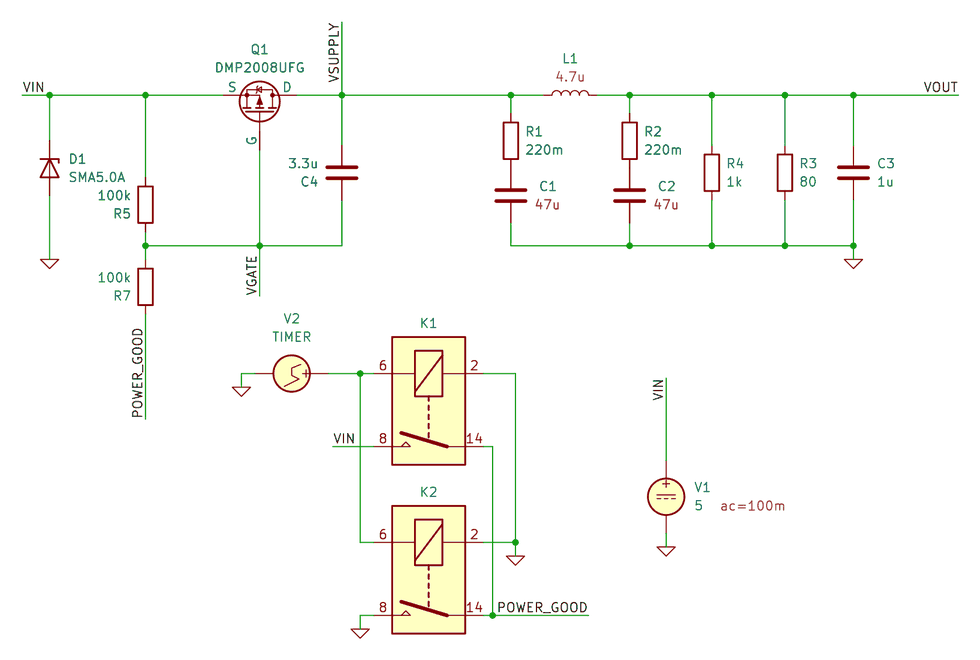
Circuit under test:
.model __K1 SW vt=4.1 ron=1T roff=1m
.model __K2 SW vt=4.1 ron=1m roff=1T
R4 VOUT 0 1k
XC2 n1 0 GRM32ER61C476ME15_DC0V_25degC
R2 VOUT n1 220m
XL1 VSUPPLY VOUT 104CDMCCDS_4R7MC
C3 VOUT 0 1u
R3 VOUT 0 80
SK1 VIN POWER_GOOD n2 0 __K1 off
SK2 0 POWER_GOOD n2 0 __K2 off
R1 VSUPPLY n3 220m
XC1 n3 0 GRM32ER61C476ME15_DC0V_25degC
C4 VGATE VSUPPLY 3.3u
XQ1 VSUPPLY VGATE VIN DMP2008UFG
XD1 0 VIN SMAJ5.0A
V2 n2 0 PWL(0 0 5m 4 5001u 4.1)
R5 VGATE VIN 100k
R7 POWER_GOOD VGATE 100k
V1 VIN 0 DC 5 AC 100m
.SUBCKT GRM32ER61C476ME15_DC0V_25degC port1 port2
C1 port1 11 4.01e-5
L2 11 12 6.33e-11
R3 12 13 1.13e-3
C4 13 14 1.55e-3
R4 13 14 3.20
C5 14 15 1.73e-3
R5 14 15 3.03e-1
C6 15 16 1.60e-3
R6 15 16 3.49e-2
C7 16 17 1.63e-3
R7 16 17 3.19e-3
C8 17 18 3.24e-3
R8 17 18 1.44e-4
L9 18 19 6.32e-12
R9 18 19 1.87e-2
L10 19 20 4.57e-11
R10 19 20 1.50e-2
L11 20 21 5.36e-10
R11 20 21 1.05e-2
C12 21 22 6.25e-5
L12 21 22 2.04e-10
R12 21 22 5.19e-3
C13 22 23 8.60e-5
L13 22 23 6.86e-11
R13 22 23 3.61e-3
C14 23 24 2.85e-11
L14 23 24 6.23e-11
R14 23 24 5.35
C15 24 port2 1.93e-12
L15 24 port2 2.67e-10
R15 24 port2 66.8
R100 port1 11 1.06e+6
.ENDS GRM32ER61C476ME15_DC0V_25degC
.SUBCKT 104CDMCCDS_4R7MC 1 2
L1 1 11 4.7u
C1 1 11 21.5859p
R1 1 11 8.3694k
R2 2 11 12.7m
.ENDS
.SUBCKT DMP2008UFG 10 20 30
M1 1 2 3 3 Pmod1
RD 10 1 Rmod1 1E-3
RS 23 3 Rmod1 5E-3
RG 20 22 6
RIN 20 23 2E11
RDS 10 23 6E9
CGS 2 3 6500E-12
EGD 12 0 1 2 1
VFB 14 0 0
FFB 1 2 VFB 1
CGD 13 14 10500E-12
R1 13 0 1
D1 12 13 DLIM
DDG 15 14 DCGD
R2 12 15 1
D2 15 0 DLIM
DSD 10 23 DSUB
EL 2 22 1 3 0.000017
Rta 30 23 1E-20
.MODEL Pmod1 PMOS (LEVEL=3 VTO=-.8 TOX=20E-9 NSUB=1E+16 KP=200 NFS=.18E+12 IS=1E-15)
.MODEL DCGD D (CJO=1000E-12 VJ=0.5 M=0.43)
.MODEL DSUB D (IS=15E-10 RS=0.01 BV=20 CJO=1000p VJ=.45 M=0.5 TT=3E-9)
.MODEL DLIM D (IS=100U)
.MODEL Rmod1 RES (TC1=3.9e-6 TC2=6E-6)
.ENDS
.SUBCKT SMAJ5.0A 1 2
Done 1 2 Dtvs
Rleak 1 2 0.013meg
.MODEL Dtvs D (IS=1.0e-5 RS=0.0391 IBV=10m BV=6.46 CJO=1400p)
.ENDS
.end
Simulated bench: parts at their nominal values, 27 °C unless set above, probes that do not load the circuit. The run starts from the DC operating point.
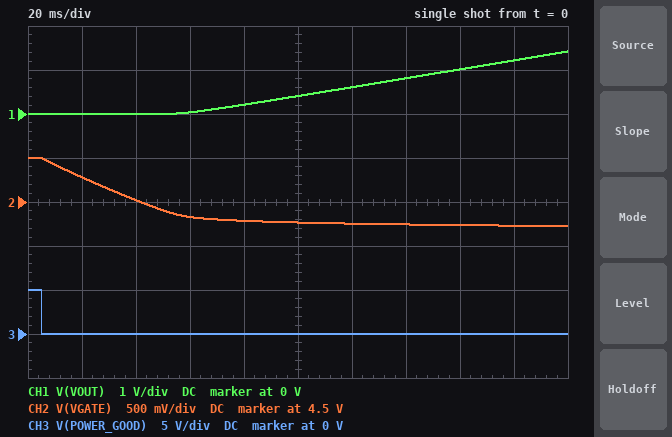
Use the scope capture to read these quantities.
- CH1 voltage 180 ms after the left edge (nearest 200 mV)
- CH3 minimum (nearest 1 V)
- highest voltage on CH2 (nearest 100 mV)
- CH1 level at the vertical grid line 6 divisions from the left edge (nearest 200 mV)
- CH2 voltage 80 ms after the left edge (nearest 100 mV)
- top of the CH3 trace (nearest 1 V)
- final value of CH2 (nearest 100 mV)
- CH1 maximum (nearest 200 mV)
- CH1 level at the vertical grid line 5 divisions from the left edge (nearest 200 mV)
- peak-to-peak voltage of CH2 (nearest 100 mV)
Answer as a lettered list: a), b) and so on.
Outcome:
a) 1.2 V
b) 0 V
c) 5.0 V
d) 600 mV
e) 4.3 V
f) 5 V
g) 4.2 V
h) 1.4 V
i) 400 mV
j) 800 mV
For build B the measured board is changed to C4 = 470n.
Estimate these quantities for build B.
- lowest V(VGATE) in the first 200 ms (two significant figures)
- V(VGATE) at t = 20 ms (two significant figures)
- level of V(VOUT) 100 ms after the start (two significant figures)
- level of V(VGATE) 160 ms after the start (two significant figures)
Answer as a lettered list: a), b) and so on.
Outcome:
a) 2.5 V
b) 4.2 V
c) 5.0 V
d) 2.6 V
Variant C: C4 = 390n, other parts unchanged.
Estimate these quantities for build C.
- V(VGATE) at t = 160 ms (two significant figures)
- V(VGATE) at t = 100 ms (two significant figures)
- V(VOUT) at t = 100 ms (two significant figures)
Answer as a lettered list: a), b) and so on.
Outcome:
a) 2.5 V
b) 2.9 V
c) 5.0 V
